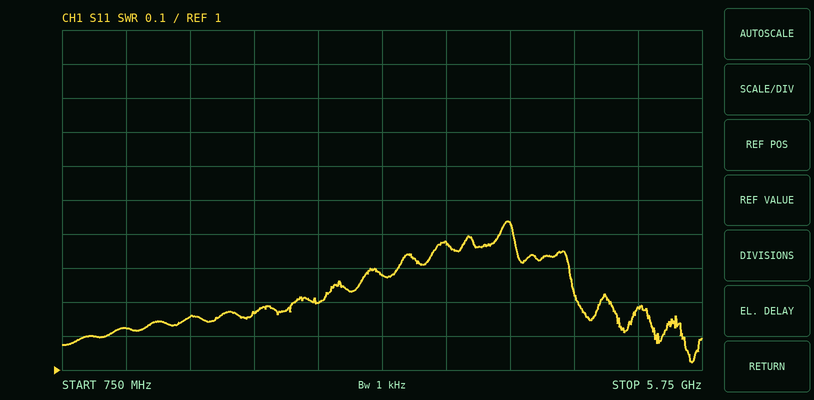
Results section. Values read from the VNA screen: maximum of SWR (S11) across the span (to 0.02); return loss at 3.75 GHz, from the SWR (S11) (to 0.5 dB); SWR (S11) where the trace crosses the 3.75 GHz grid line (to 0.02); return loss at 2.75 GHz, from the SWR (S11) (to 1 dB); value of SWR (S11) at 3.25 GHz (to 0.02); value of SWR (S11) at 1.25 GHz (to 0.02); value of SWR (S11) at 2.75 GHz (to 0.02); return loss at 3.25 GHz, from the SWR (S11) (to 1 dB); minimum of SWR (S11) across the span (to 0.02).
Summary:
1.44
16.0 dB
1.38
21 dB
1.28
1.12
1.20
18 dB
1.02
